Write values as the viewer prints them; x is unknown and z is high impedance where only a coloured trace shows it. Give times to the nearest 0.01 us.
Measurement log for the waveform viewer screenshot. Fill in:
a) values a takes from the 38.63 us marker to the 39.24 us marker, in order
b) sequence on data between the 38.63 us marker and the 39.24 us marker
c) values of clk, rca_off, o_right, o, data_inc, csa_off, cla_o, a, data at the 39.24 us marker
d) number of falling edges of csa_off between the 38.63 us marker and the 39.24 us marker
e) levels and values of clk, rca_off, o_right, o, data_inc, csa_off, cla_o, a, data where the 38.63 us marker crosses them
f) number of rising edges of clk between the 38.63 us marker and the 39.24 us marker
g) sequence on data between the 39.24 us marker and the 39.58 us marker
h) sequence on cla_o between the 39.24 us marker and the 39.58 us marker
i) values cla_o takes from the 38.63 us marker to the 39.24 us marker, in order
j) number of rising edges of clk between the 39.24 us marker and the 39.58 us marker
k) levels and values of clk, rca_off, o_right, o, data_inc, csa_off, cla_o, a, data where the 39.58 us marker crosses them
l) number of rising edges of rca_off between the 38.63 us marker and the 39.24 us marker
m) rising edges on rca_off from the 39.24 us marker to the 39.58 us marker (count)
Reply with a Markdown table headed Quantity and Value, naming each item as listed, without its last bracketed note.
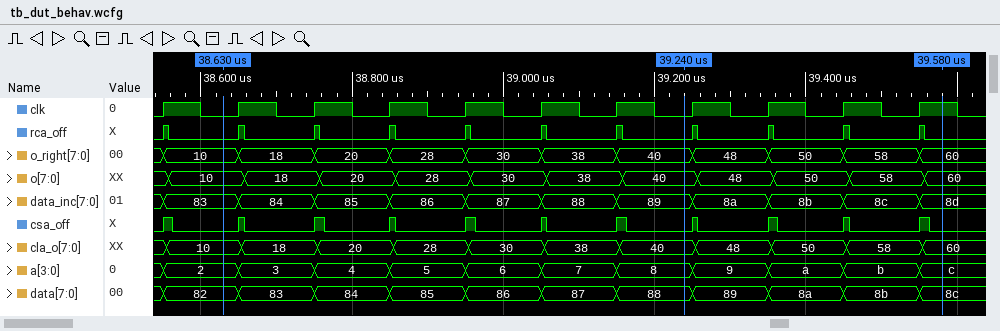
| Quantity | Value |
|---|---|
| values a takes from the 38.63 us marker to the 39.24 us marker, in order | 2, 3, 4, 5, 6, 7, 8 |
| sequence on data between the 38.63 us marker and the 39.24 us marker | 82, 83, 84, 85, 86, 87, 88 |
| values of clk, rca_off, o_right, o, data_inc, csa_off, cla_o, a, data at the 39.24 us marker | clk=0, rca_off=0, o_right=40, o=40, data_inc=89, csa_off=0, cla_o=40, a=8, data=88 |
| number of falling edges of csa_off between the 38.63 us marker and the 39.24 us marker | 6 |
| levels and values of clk, rca_off, o_right, o, data_inc, csa_off, cla_o, a, data where the 38.63 us marker crosses them | clk=0, rca_off=0, o_right=10, o=10, data_inc=83, csa_off=0, cla_o=10, a=2, data=82 |
| number of rising edges of clk between the 38.63 us marker and the 39.24 us marker | 6 |
| sequence on data between the 39.24 us marker and the 39.58 us marker | 88, 89, 8a, 8b, 8c |
| sequence on cla_o between the 39.24 us marker and the 39.58 us marker | 40, 48, 50, 58, 60 |
| values cla_o takes from the 38.63 us marker to the 39.24 us marker, in order | 10, 18, 20, 28, 30, 38, 40 |
| number of rising edges of clk between the 39.24 us marker and the 39.58 us marker | 4 |
| levels and values of clk, rca_off, o_right, o, data_inc, csa_off, cla_o, a, data where the 39.58 us marker crosses them | clk=1, rca_off=0, o_right=60, o=60, data_inc=8d, csa_off=0, cla_o=60, a=c, data=8c |
| number of rising edges of rca_off between the 38.63 us marker and the 39.24 us marker | 6 |
| rising edges on rca_off from the 39.24 us marker to the 39.58 us marker | 4 |
